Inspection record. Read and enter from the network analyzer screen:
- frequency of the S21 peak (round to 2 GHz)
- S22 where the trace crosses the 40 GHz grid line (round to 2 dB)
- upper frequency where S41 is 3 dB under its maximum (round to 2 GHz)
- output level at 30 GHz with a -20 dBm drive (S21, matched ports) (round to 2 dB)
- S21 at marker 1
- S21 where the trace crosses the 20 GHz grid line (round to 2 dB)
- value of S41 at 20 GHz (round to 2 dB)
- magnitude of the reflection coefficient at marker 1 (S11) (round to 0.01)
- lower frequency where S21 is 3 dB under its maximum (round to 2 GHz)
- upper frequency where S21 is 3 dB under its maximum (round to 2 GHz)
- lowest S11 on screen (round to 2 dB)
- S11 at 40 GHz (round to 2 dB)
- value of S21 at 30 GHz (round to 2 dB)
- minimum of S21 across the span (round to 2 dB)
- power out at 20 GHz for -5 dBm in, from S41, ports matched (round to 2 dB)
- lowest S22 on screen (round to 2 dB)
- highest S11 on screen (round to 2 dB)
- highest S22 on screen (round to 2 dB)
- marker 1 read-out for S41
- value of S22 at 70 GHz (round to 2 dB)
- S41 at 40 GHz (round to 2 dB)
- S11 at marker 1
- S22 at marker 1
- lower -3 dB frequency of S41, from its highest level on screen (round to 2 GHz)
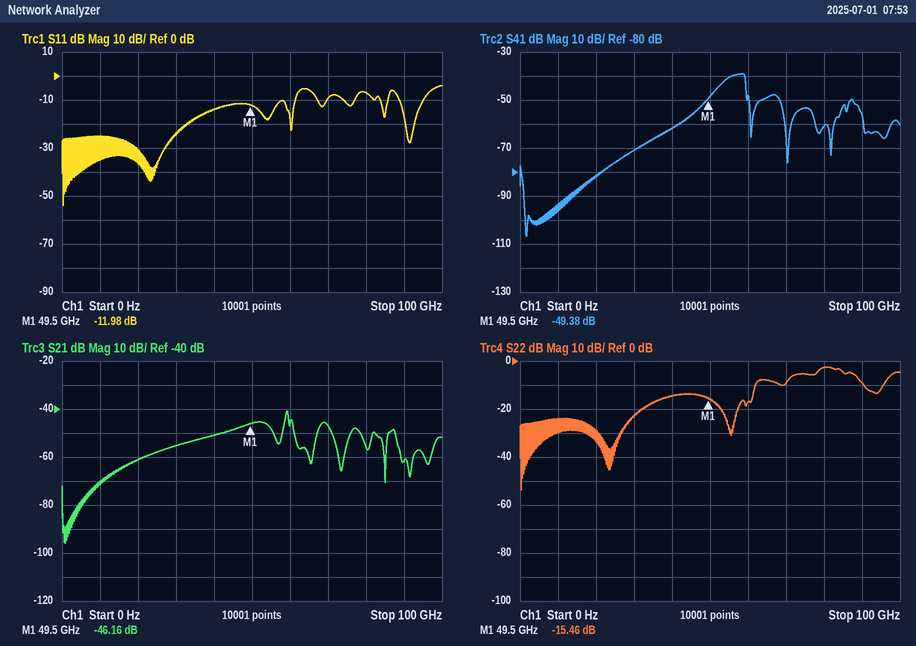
60 GHz
-14 dB
60 GHz
-76 dBm
-46.16 dB
-62 dB
-82 dB
0.25
58 GHz
60 GHz
-54 dB
-14 dB
-56 dB
-96 dB
-86 dBm
-54 dB
-4 dB
-2 dB
-49.38 dB
-10 dB
-62 dB
-11.98 dB
-15.46 dB
54 GHz
